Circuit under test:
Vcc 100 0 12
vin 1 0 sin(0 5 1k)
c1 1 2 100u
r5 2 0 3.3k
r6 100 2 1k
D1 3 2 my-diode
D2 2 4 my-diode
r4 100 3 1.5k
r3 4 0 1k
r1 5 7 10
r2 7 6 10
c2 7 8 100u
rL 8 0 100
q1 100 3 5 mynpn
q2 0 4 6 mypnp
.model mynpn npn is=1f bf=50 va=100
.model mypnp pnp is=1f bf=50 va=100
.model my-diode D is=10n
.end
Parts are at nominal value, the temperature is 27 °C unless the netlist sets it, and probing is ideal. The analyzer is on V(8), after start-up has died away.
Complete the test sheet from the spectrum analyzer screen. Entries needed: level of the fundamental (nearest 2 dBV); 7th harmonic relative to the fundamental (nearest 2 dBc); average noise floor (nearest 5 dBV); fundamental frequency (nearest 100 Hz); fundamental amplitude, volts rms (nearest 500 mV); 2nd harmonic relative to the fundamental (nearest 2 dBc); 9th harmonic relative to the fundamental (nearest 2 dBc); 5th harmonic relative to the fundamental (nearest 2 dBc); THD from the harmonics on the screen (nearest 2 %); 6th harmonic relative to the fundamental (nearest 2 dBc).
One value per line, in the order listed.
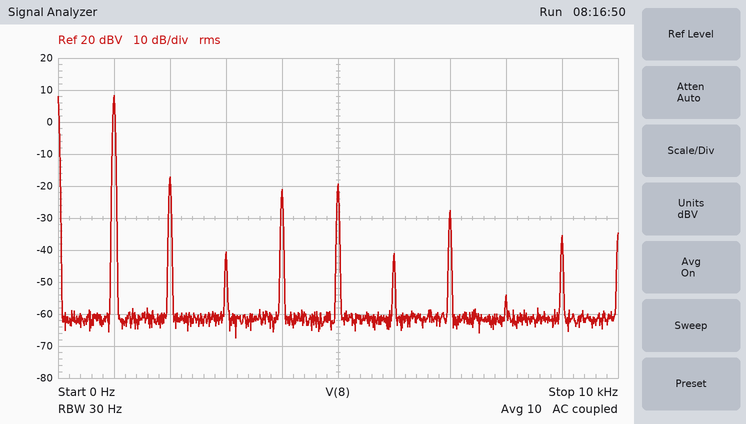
8 dBV
-36 dBc
-60 dBV
1.0 kHz
2.5 V
-26 dBc
-44 dBc
-28 dBc
8 %
-50 dBc
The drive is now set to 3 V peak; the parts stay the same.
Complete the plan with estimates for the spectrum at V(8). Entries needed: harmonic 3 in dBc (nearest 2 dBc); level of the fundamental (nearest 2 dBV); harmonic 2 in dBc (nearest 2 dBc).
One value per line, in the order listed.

-24 dBc
4 dBV
-58 dBc
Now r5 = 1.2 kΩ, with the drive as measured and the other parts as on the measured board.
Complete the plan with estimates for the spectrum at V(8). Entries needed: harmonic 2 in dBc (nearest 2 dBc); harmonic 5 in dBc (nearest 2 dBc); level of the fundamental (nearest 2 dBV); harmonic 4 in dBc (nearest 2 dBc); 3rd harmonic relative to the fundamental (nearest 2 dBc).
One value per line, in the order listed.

-46 dBc
-30 dBc
8 dBV
-48 dBc
-32 dBc
